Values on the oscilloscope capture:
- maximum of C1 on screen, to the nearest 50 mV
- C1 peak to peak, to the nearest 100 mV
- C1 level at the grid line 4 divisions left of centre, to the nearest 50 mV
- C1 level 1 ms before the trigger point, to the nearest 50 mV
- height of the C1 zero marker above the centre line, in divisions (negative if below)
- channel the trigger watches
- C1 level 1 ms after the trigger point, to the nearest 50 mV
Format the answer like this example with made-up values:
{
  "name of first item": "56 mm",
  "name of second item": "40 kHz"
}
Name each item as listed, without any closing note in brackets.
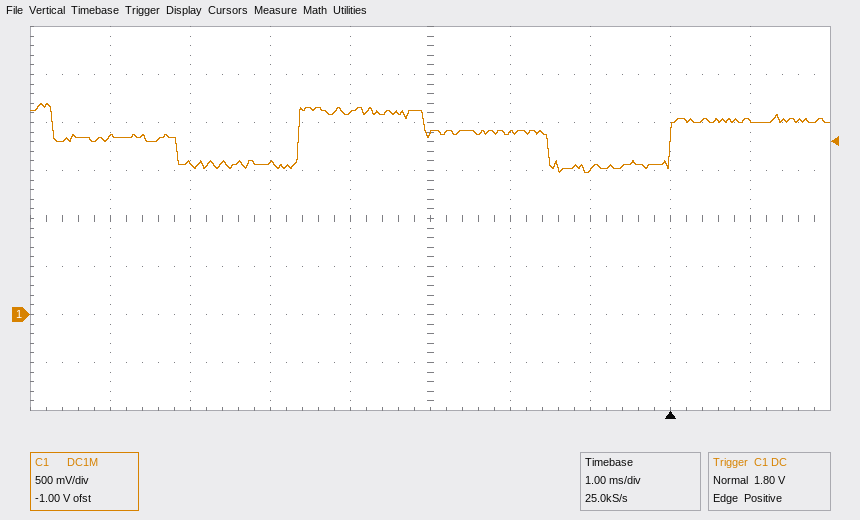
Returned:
{
  "maximum of C1 on screen, to the nearest 50 mV": "2.20 V",
  "C1 peak to peak, to the nearest 100 mV": "700 mV",
  "C1 level at the grid line 4 divisions left of centre, to the nearest 50 mV": "1.85 V",
  "C1 level 1 ms before the trigger point, to the nearest 50 mV": "1.50 V",
  "height of the C1 zero marker above the centre line, in divisions": "-2.0 div",
  "channel the trigger watches": "C1",
  "C1 level 1 ms after the trigger point, to the nearest 50 mV": "2.00 V"
}
